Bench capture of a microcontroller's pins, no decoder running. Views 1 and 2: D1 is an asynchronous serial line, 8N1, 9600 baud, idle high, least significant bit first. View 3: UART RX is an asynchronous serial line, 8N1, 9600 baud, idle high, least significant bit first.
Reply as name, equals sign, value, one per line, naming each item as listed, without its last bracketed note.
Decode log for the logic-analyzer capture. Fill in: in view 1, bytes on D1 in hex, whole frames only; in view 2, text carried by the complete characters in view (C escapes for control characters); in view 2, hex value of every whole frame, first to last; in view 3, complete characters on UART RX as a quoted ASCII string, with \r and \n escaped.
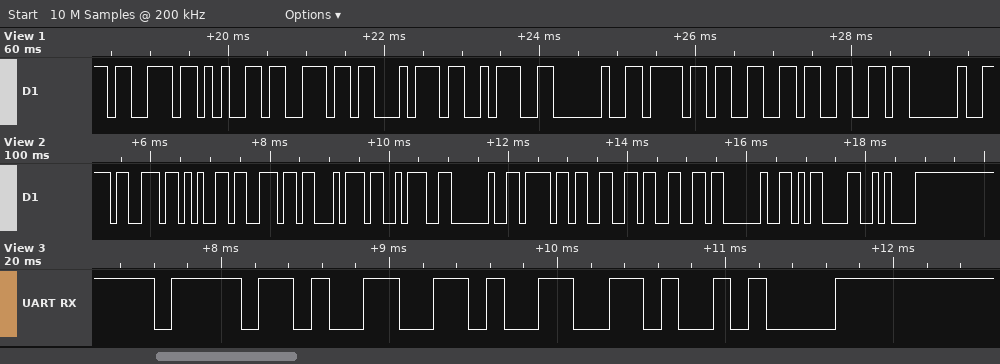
in view 1, bytes on D1 in hex, whole frames only = 0x73 0x65 0x6E 0x74 0x3A 0x20 0x6F 0x66 0x66 0x20
in view 2, text carried by the complete characters in view = "sent: off \r\n"
in view 2, hex value of every whole frame, first to last = 0x73 0x65 0x6E 0x74 0x3A 0x20 0x6F 0x66 0x66 0x20 0x0D 0x0A
in view 3, complete characters on UART RX as a quoted ASCII string, with \r and \n escaped = "off\n"
